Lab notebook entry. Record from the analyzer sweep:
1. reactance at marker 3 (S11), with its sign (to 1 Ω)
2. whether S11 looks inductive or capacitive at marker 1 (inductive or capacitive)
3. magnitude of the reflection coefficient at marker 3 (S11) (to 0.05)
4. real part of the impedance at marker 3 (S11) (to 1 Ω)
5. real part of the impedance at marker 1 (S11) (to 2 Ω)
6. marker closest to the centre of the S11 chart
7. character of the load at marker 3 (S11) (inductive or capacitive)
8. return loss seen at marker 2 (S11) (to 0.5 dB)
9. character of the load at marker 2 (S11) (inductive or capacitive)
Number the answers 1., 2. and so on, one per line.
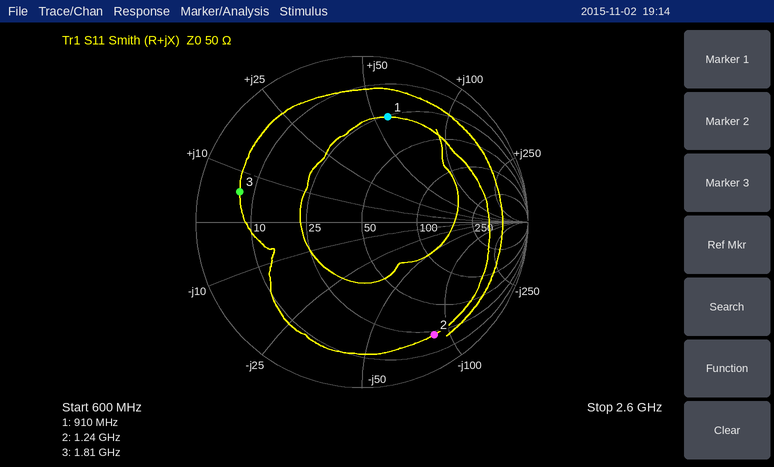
1. +6 Ω
2. inductive
3. 0.75
4. 7 Ω
5. 26 Ω
6. marker 1
7. inductive
8. 2.0 dB
9. capacitive
